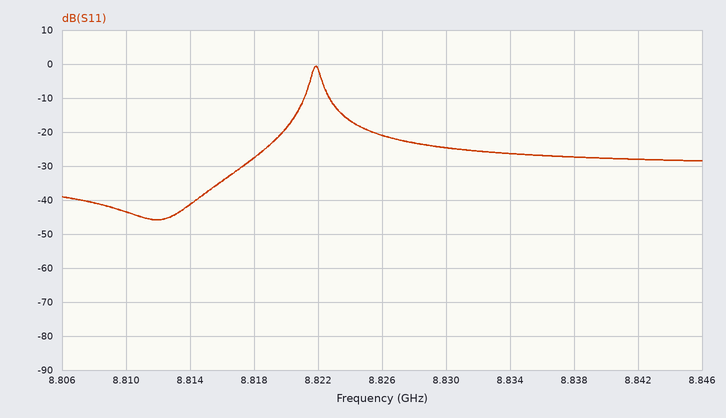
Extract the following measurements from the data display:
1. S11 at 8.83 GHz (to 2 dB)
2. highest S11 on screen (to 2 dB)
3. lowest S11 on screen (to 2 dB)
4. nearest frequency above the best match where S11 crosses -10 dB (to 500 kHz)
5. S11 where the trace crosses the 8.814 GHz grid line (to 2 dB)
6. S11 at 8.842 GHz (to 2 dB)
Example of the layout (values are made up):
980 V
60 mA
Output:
-24 dB
0 dB
-46 dB
8.8210 GHz
-42 dB
-28 dB
